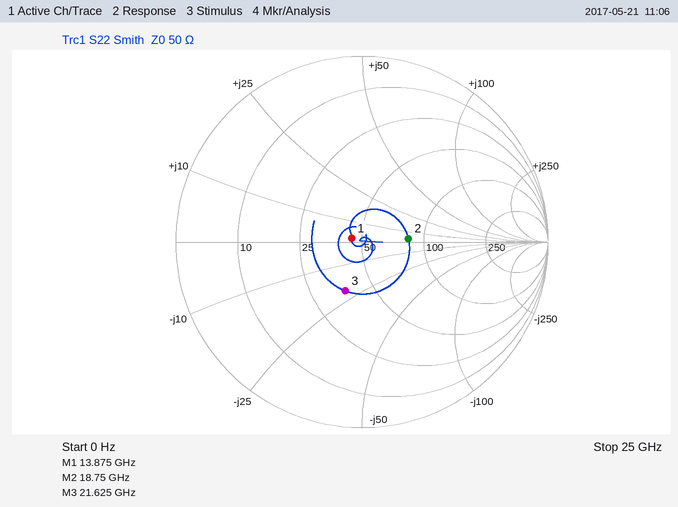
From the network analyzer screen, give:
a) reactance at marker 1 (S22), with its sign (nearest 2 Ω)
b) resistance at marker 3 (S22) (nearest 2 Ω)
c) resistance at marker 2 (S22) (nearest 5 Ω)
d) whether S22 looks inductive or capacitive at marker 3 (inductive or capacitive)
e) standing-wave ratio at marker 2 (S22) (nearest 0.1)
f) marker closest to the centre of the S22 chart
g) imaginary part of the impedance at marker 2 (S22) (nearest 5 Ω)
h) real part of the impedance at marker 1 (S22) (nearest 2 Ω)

+2 Ω
36 Ω
85 Ω
capacitive
1.7
marker 1
+5 Ω
44 Ω
